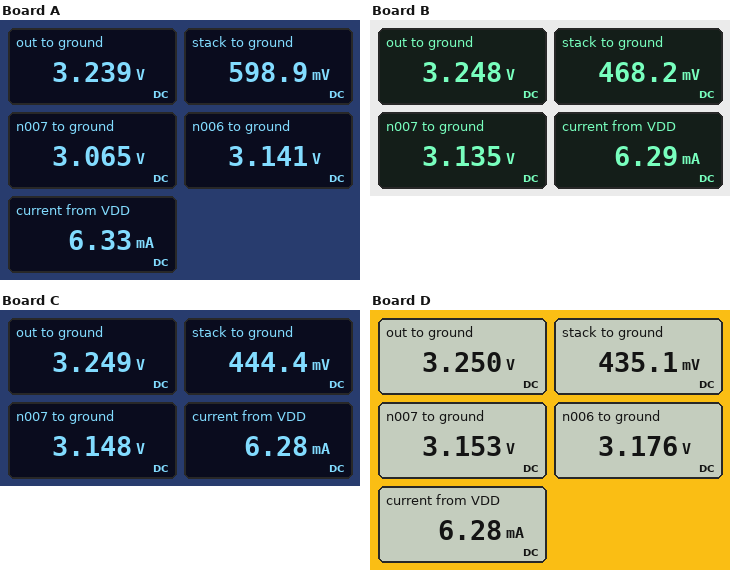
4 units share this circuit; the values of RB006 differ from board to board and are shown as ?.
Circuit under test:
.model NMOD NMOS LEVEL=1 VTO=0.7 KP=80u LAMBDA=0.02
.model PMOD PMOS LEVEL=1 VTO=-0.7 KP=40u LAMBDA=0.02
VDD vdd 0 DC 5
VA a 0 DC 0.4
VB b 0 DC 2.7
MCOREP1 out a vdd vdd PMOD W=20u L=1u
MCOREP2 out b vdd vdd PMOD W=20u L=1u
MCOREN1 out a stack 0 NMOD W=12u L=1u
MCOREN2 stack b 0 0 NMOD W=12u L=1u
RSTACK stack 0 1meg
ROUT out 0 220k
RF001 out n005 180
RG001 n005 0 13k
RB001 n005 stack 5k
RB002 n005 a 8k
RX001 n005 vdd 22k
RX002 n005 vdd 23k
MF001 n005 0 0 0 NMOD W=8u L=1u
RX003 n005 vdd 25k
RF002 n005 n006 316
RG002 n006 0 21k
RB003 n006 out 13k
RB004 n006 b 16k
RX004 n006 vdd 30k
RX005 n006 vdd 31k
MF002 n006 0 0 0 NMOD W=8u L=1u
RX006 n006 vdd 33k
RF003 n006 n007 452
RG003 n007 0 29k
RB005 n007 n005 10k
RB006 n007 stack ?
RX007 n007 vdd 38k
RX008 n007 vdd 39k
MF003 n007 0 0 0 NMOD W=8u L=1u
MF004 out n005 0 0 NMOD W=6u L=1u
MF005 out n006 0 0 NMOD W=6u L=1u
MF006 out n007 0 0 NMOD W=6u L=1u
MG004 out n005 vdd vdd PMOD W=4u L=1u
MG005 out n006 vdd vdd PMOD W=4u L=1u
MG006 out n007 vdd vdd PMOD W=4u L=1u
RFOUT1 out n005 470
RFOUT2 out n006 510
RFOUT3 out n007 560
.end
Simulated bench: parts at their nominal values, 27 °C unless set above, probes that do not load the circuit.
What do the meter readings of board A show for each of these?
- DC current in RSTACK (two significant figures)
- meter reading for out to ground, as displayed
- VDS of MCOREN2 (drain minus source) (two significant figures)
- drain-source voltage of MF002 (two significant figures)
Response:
600 nA
3.239 V
600 mV
3.1 V
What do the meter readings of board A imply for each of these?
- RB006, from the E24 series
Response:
5.1 kΩ
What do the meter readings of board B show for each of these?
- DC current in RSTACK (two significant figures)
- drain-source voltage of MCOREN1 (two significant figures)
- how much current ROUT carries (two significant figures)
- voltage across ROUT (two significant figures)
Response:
470 nA
2.8 V
15 µA
3.2 V
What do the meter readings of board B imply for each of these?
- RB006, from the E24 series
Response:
10 kΩ
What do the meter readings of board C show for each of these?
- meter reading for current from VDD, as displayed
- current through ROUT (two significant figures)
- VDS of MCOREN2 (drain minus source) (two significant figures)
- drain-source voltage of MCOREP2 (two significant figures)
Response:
6.28 mA
15 µA
440 mV
-1.8 V
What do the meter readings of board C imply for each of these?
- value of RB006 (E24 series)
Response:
12 kΩ
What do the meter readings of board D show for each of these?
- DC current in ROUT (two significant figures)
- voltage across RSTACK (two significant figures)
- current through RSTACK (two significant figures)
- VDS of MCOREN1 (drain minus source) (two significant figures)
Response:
15 µA
440 mV
440 nA
2.8 V
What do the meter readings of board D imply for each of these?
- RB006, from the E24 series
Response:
13 kΩ
